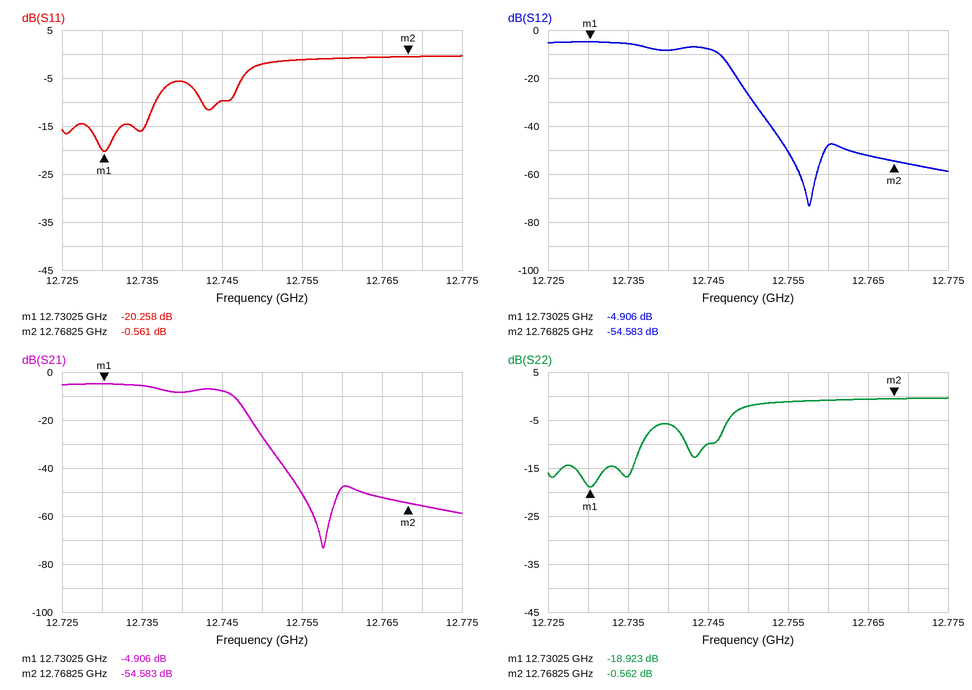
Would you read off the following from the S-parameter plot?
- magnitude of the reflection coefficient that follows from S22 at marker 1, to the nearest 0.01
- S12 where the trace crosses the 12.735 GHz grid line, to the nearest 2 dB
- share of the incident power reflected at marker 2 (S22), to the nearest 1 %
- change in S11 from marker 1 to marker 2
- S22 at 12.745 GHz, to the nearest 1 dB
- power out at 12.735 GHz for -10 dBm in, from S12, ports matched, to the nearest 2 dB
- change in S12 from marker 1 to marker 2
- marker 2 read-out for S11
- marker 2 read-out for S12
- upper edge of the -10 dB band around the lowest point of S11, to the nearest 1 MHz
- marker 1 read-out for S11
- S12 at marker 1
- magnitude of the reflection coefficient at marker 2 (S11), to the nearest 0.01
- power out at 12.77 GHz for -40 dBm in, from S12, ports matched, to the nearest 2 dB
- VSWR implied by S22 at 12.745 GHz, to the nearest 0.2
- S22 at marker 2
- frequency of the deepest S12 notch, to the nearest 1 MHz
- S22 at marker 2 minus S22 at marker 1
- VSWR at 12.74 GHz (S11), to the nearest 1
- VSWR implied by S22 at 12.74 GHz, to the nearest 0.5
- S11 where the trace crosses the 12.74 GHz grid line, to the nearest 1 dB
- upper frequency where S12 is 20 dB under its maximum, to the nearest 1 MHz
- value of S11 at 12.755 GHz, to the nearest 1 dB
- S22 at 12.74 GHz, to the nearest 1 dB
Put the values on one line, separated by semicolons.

0.11; -6 dB; 88 %; 19.697 dB; -10 dB; -16 dBm; -49.677 dB; -0.561 dB; -54.583 dB; 12.737 GHz; -20.258 dB; -4.906 dB; 0.94; -96 dBm; 2.0; -0.562 dB; 12.758 GHz; 18.361 dB; 3; 3.0; -6 dB; 12.750 GHz; -1 dB; -6 dB
